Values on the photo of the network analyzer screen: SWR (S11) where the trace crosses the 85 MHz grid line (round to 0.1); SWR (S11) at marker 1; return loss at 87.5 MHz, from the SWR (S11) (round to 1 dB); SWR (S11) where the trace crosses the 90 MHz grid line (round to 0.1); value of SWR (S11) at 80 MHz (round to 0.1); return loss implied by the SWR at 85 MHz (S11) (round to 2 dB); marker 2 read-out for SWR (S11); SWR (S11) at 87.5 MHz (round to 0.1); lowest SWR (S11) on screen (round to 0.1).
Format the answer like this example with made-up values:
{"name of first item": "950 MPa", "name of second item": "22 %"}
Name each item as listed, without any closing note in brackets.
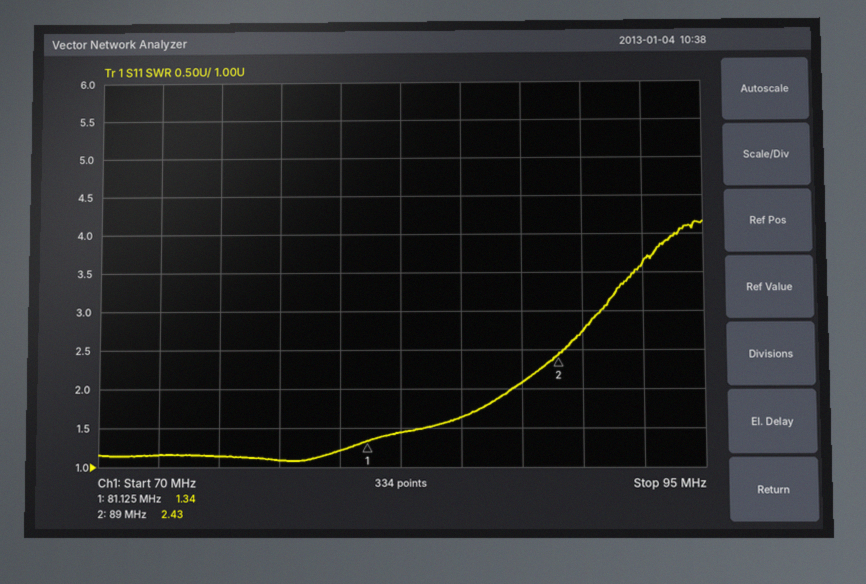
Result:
{"SWR (S11) where the trace crosses the 85 MHz grid line": "1.6", "SWR (S11) at marker 1": "1.34", "return loss at 87.5 MHz, from the SWR (S11)": "9 dB", "SWR (S11) where the trace crosses the 90 MHz grid line": "2.7", "value of SWR (S11) at 80 MHz": "1.2", "return loss implied by the SWR at 85 MHz (S11)": "12 dB", "marker 2 read-out for SWR": "2.43", "SWR (S11) at 87.5 MHz": "2.1", "lowest SWR (S11) on screen": "1.1"}
